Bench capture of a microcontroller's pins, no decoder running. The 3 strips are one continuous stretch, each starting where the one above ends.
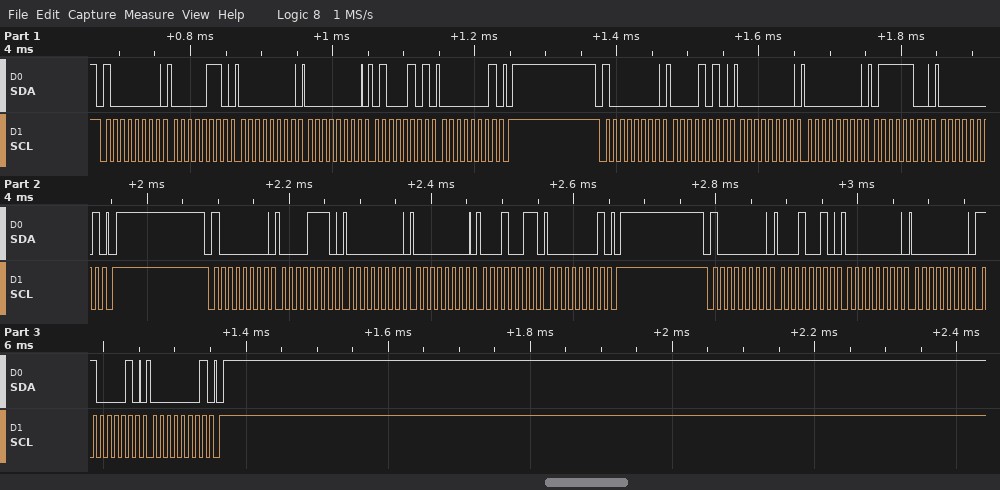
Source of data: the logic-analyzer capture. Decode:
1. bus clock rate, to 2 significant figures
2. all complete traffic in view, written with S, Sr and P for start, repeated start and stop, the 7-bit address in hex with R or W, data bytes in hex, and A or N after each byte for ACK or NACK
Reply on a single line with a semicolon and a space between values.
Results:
100 kHz; S 40W A 06 A 00 A 00 A 45 A 01 A P S 40W A 0A A 00 A 00 A 7C A 01 A P S 40W A 0E A 00 A 00 A 13 A 01 A P S 40W A 12 A 00 A 00 A C2 A 01 A P
